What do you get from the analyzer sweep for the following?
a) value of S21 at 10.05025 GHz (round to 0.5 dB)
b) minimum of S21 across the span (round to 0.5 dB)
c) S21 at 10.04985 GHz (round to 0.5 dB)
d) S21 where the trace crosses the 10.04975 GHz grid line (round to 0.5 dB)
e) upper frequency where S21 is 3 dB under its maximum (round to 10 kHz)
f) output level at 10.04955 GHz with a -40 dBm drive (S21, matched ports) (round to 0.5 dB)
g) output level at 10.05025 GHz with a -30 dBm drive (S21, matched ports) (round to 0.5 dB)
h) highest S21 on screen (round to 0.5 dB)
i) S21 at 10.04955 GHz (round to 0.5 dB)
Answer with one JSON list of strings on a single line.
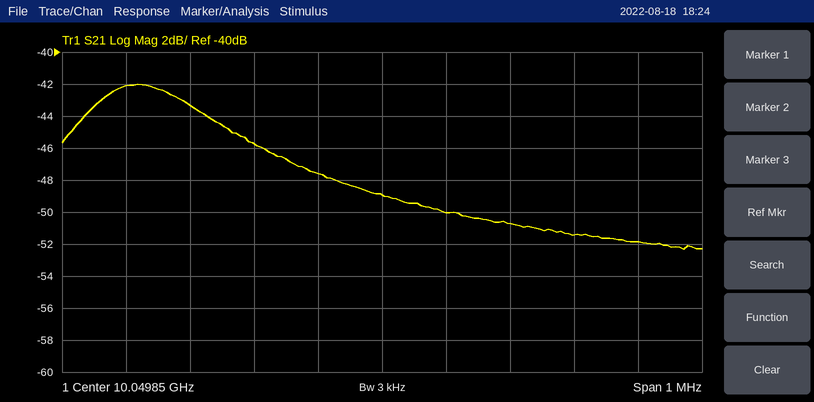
["-52.0 dB", "-52.5 dB", "-49.0 dB", "-47.5 dB", "10.04962 GHz", "-83.5 dBm", "-82.0 dBm", "-42.0 dB", "-43.5 dB"]
